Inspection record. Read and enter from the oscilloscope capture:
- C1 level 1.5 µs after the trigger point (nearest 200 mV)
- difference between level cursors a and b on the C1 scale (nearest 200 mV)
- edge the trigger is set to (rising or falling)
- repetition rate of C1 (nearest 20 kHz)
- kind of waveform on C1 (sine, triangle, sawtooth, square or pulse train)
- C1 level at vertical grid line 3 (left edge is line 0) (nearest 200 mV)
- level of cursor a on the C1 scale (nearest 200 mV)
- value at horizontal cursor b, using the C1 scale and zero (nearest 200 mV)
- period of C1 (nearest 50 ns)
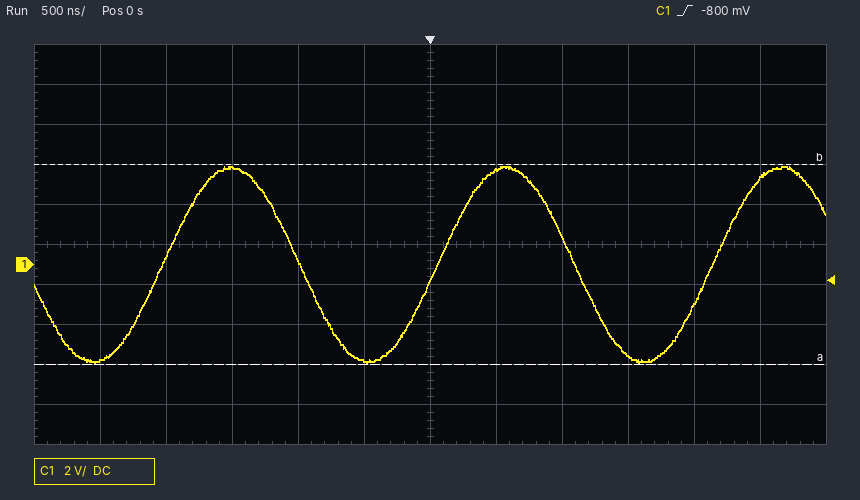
-4.6 V
10.0 V
rising
480 kHz
sine
4.8 V
-5.0 V
5.0 V
2.10 µs
